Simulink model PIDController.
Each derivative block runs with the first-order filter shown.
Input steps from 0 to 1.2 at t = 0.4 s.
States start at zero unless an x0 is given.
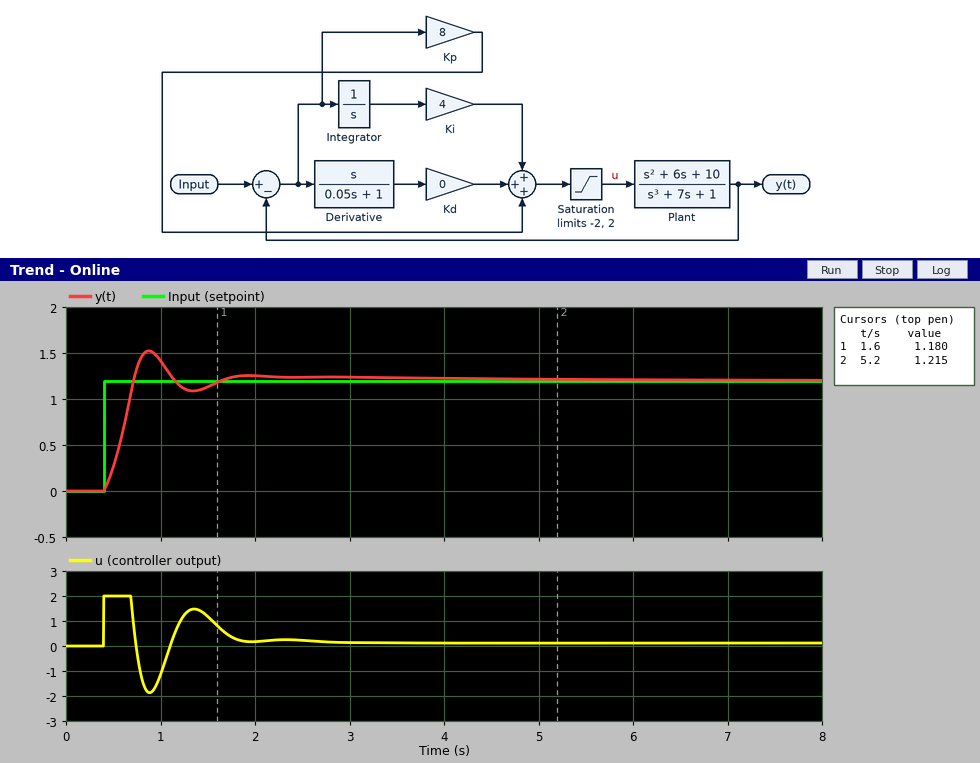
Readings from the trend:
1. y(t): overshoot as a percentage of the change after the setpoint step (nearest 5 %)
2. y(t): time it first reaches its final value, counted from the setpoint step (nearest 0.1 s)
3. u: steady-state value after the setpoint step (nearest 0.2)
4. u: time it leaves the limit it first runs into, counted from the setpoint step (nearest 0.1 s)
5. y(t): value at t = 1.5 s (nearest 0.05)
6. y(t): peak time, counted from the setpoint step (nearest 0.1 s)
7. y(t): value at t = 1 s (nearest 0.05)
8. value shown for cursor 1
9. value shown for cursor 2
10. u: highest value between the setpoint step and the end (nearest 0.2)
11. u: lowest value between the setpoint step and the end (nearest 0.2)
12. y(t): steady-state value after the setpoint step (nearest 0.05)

25 %
0.3 s
0.2
0.3 s
1.15
0.5 s
1.40
1.180
1.215
2.0
-1.8
1.20
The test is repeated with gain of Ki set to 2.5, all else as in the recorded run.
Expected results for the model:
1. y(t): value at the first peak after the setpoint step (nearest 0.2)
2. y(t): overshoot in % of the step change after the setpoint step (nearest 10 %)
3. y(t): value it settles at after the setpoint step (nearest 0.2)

1.4
20 %
1.2
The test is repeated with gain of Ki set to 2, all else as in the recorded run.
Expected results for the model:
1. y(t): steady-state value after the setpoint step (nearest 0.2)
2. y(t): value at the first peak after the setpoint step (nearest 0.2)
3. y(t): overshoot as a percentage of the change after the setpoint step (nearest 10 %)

1.2
1.4
20 %
